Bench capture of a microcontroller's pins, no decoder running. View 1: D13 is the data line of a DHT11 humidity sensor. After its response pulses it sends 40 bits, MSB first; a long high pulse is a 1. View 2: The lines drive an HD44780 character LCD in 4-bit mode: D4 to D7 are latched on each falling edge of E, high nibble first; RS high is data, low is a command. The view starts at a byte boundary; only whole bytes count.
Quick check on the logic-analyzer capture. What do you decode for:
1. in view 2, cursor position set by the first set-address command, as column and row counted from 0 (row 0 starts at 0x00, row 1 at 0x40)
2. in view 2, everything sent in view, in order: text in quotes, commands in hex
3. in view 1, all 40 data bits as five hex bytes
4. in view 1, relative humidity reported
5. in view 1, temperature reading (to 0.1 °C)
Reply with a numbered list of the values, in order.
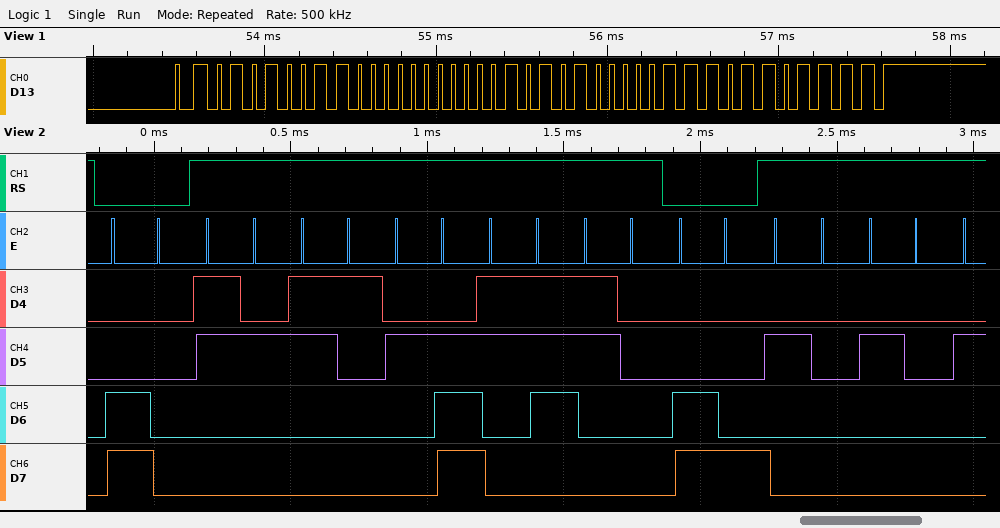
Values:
1. column 0, row 1
2. 0xC0 "21.70" 0xC8 "  "
3. 53 00 15 07 6F
4. 83 %
5. 21.7 °C
